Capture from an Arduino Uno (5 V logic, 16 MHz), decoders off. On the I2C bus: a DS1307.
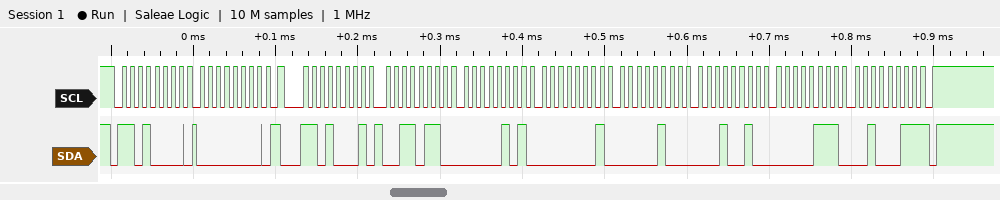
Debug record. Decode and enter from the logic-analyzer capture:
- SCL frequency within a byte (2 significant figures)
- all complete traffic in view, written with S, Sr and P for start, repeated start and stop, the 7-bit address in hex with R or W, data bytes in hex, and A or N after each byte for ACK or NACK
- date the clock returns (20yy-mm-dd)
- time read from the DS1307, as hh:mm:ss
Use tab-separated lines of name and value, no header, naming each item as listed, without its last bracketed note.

SCL frequency within a byte	100 kHz
all complete traffic in view, written with S, Sr and P for start, repeated start and stop, the 7-bit address in hex with R or W, data bytes in hex, and A or N after each byte for ACK or NACK	S 68W A 00 A Sr 68R A 36 A 05 A 01 A 04 A 12 A 07 A 23 N P
date the clock returns	2023-07-12
time read from the DS1307, as hh:mm:ss	01:05:36
